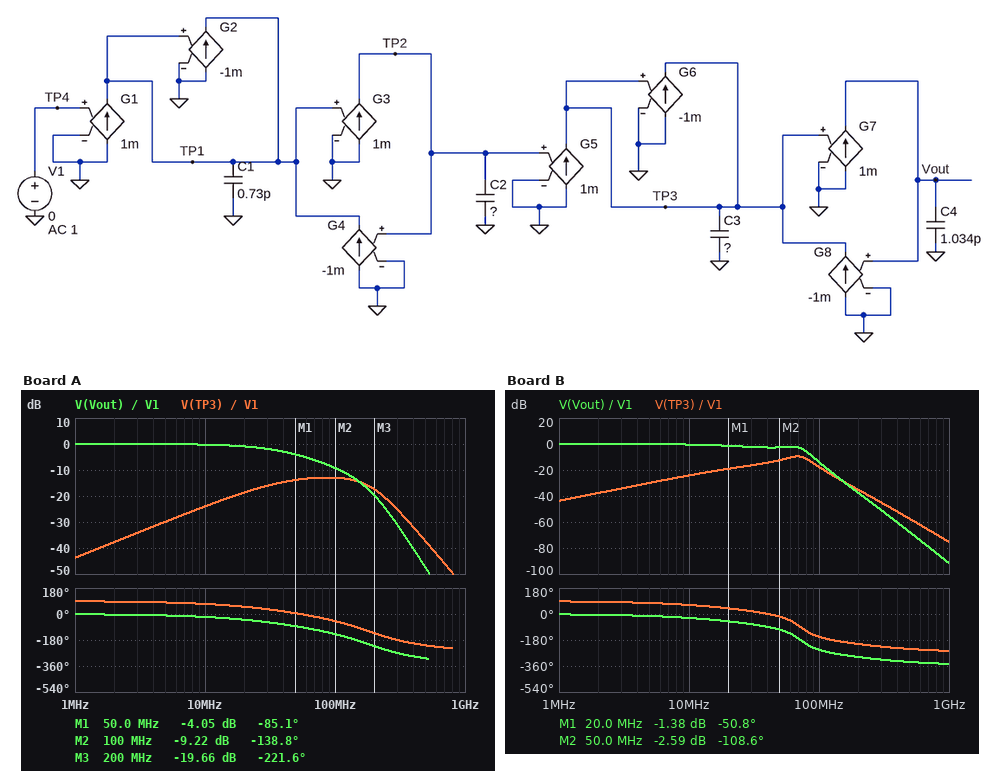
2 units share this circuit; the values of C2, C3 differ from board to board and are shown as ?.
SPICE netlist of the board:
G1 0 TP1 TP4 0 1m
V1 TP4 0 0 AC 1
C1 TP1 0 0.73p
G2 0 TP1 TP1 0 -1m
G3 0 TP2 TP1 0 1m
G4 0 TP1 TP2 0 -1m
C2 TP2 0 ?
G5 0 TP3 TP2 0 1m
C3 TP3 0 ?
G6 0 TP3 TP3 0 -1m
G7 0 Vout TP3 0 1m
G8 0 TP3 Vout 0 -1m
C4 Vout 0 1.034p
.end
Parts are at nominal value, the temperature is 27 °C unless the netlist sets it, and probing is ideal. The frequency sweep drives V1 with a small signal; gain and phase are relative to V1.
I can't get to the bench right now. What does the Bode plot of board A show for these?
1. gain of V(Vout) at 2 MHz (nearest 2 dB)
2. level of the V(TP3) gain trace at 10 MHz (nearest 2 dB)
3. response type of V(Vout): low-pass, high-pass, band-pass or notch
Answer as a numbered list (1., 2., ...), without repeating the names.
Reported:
1. 0 dB
2. -24 dB
3. low-pass
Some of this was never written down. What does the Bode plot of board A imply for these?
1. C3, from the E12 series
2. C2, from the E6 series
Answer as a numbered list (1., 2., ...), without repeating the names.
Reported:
1. 680 fF
2. 4.7 pF
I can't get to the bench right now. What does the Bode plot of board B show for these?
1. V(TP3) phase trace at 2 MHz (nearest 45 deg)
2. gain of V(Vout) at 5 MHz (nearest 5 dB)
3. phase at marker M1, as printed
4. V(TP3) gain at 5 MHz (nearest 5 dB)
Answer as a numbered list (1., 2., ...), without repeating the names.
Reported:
1. 90 deg
2. 0 dB
3. -50.8 deg
4. -30 dB
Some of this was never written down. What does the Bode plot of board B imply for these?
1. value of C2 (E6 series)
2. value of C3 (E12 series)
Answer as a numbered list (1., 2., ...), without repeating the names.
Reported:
1. 6.8 pF
2. 4.7 pF
